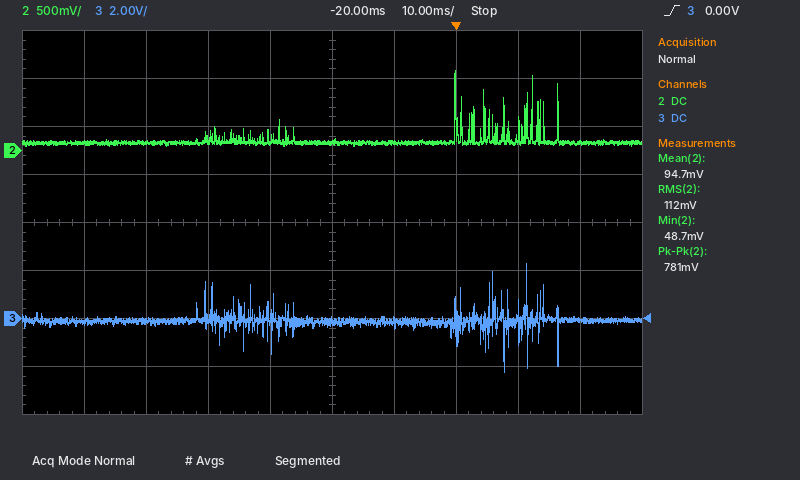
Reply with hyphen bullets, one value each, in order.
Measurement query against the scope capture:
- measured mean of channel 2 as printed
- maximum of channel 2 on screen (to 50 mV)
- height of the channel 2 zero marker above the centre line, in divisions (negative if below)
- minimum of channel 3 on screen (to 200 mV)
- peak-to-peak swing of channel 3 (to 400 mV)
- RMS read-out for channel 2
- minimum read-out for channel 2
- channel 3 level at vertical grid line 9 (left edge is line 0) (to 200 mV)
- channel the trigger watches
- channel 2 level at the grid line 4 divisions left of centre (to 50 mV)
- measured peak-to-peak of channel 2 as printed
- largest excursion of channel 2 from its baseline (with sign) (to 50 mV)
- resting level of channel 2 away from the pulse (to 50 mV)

- 94.7 mV
- 850 mV
- +1.5 div
- -2.2 V
- 4.4 V
- 112 mV
- 48.7 mV
- 0.0 V
- channel 3
- 100 mV
- 781 mV
- +750 mV
- 100 mV
